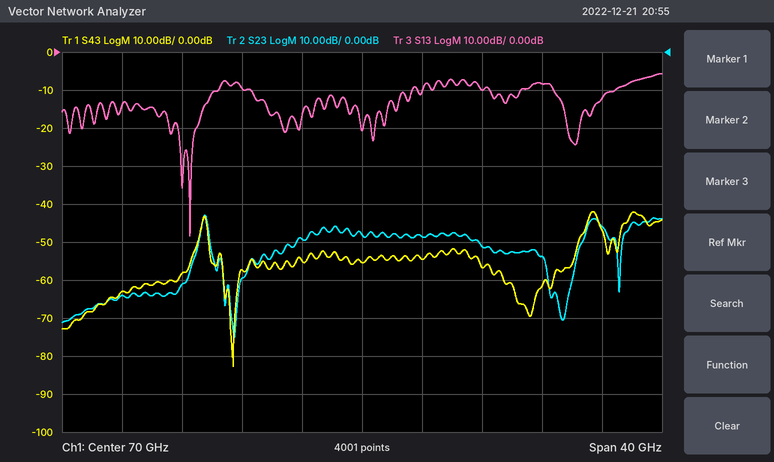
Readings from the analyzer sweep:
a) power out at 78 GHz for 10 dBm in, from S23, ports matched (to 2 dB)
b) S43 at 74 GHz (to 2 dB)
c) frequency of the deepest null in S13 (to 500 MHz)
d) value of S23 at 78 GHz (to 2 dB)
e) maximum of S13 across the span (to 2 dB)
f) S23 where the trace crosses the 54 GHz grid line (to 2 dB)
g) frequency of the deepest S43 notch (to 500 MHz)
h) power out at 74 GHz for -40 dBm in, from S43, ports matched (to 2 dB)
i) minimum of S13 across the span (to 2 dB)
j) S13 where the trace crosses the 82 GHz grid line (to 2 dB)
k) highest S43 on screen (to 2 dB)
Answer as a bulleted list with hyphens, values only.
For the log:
- -42 dBm
- -54 dB
- 58.5 GHz
- -52 dB
- -6 dB
- -64 dB
- 61.5 GHz
- -94 dBm
- -48 dB
- -8 dB
- -42 dB
